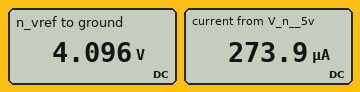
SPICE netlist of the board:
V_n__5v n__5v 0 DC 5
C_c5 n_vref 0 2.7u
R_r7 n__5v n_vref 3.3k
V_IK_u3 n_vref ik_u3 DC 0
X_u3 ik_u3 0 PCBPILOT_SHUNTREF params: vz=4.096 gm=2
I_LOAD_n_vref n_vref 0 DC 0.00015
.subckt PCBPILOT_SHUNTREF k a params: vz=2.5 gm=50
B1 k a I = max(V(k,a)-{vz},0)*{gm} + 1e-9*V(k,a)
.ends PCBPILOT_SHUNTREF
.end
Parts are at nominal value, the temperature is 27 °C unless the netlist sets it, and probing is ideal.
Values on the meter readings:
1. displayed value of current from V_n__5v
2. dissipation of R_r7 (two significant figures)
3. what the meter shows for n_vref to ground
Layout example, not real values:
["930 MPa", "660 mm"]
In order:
["273.9 µA", "250 µW", "4.096 V"]
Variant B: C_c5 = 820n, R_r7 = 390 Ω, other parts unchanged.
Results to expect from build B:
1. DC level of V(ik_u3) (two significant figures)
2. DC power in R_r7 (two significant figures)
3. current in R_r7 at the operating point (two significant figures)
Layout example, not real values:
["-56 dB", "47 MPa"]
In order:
["4.1 V", "2.1 mW", "2.3 mA"]
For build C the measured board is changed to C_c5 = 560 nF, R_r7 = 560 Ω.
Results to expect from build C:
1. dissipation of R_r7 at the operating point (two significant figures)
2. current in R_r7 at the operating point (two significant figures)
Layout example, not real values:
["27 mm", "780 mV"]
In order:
["1.5 mW", "1.6 mA"]
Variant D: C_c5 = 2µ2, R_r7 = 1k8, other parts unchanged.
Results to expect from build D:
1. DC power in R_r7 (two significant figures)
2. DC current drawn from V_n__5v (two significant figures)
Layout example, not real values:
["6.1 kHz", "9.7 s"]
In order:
["450 µW", "500 µA"]
